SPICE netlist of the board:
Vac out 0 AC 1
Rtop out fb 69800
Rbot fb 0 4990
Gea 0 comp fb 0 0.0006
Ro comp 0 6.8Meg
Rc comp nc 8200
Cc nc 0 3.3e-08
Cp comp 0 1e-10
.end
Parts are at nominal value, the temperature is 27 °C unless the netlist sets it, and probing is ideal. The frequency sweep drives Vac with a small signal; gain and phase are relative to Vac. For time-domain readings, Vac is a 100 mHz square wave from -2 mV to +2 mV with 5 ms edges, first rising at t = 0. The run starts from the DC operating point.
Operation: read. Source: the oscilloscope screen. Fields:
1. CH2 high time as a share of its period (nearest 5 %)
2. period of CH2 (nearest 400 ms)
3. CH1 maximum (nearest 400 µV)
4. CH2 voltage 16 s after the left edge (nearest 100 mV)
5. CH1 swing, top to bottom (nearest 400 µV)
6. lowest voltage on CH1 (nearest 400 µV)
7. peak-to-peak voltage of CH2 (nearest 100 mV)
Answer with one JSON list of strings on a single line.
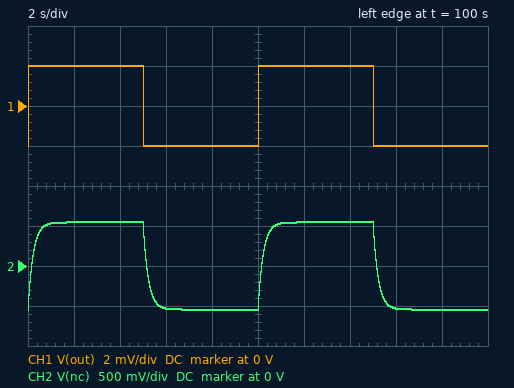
["50 %", "10.0 s", "2.0 mV", "-500 mV", "4.0 mV", "-2.0 mV", "1.1 V"]
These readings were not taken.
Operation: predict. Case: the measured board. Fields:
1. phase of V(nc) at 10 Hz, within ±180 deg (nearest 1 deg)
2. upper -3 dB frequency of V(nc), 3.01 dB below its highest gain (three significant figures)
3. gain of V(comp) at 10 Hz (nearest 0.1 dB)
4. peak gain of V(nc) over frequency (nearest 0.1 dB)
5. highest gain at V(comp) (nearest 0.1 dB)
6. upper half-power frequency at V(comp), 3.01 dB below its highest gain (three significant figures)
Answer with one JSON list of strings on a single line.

["-86 deg", "706 mHz", "25.7 dB", "48.7 dB", "48.7 dB", "706 mHz"]
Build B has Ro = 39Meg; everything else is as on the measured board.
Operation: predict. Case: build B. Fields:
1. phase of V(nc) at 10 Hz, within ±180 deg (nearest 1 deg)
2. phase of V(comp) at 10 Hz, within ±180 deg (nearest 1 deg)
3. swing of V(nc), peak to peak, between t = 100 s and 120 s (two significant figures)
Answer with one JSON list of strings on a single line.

["-89 deg", "-88 deg", "6.0 V"]
